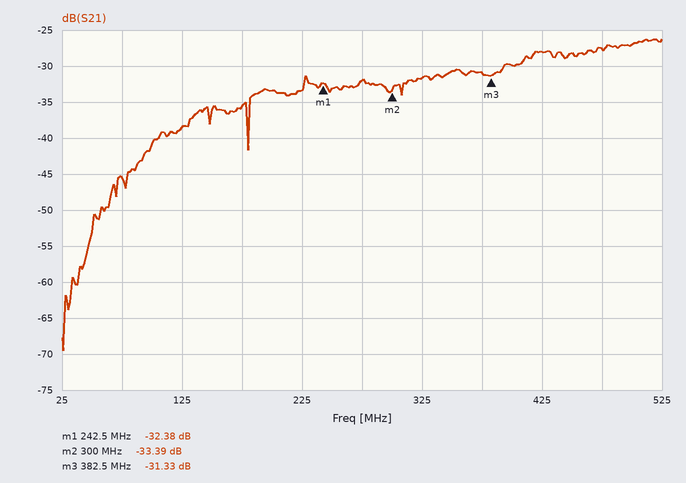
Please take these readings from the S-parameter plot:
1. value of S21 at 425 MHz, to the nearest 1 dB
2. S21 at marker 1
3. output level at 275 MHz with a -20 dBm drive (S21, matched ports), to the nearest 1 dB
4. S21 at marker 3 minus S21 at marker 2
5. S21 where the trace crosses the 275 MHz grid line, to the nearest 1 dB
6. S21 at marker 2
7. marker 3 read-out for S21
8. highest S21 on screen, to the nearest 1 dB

-28 dB
-32.38 dB
-52 dBm
2.06 dB
-32 dB
-33.39 dB
-31.33 dB
-26 dB
